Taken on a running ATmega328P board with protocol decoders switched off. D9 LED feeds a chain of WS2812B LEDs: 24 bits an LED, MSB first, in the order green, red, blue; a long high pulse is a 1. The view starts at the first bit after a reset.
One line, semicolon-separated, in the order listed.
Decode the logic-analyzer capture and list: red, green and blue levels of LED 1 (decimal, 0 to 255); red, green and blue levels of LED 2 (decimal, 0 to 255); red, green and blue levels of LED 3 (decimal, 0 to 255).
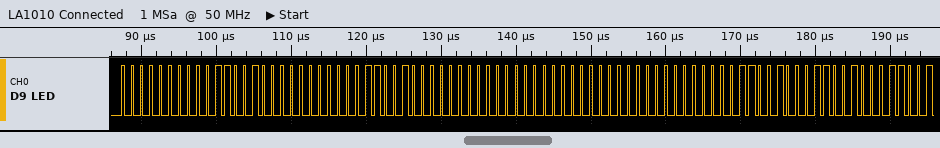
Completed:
50, 0, 0; 0, 50, 0; 0, 0, 50
